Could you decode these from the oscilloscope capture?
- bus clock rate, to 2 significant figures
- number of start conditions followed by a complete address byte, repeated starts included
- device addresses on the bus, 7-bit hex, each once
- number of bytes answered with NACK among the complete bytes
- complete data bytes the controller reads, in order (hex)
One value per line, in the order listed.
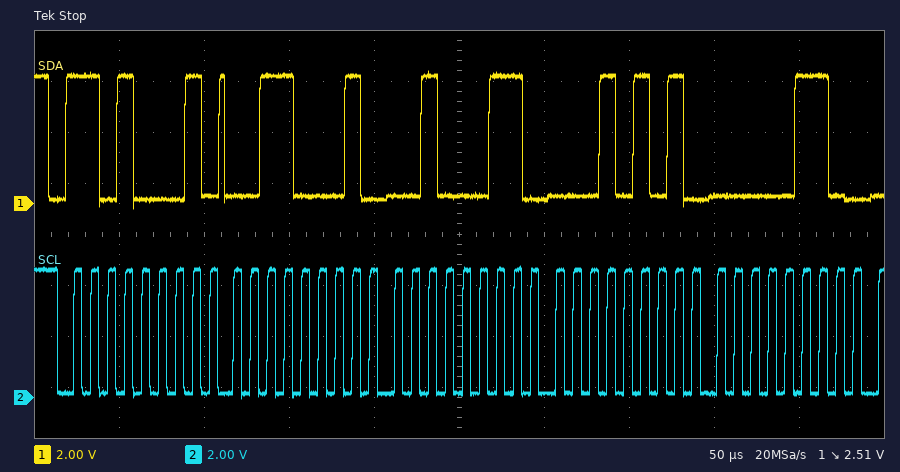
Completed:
100 kHz
1
0x68
0
31 23 15 06
